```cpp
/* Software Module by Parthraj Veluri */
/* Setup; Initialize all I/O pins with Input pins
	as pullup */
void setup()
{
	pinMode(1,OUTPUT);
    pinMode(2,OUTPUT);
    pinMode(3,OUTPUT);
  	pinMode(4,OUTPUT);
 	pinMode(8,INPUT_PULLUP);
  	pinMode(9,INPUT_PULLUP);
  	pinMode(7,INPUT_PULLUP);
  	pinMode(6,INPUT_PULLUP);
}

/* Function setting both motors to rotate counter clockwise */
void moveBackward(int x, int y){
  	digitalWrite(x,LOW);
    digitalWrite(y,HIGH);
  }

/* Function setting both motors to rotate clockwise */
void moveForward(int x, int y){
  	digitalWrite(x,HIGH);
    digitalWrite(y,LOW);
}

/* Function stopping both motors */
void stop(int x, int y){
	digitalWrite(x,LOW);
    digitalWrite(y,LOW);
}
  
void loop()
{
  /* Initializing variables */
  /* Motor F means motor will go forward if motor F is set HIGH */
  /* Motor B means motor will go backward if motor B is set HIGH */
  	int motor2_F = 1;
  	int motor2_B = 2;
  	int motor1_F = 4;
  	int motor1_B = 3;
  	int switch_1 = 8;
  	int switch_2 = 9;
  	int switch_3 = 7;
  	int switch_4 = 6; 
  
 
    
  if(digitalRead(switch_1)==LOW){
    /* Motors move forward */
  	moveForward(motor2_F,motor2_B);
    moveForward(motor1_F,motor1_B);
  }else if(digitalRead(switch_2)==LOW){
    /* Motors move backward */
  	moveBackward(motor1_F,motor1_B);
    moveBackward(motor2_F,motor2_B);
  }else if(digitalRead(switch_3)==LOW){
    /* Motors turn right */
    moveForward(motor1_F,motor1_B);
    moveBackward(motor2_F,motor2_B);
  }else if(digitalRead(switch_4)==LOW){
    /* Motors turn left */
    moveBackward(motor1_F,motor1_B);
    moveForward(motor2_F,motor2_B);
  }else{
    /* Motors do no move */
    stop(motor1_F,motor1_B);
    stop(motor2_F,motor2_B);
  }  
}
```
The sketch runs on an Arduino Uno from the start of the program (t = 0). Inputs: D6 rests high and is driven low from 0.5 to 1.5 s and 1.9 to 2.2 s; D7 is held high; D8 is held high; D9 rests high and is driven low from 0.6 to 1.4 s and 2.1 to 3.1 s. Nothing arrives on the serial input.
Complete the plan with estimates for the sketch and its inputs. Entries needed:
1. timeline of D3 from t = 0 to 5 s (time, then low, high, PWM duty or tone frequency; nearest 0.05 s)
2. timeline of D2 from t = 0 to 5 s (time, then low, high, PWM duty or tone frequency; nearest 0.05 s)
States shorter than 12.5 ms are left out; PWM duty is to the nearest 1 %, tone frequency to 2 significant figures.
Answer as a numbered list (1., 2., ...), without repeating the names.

1. 0 s low; 0.5 s high; 1.5 s low; 1.9 s high; 3.1 s low
2. 0 s low; 0.6 s high; 1.4 s low; 2.1 s high; 3.1 s low
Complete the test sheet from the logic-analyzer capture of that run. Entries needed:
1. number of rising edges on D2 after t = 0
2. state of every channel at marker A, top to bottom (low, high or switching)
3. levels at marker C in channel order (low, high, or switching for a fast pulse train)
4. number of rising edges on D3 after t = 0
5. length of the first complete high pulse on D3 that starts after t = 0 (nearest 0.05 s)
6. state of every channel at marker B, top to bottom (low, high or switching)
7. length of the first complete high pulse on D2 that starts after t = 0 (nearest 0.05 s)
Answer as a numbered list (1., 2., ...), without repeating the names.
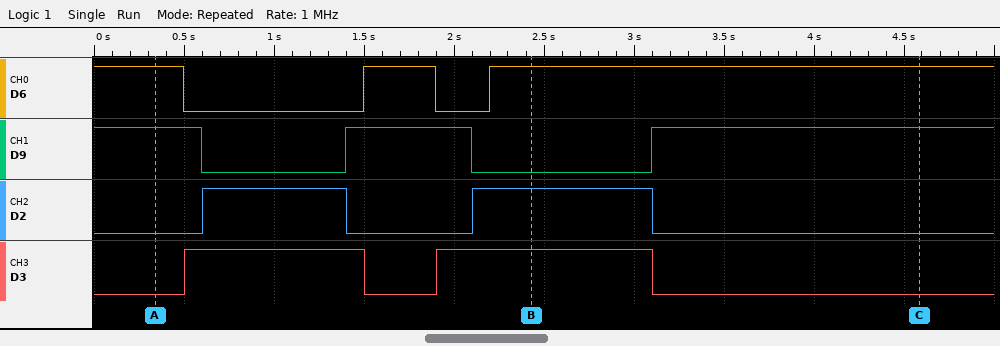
1. 2
2. D6 high, D9 high, D2 low, D3 low
3. D6 high, D9 high, D2 low, D3 low
4. 2
5. 1.00 s
6. D6 high, D9 low, D2 high, D3 high
7. 0.80 s
